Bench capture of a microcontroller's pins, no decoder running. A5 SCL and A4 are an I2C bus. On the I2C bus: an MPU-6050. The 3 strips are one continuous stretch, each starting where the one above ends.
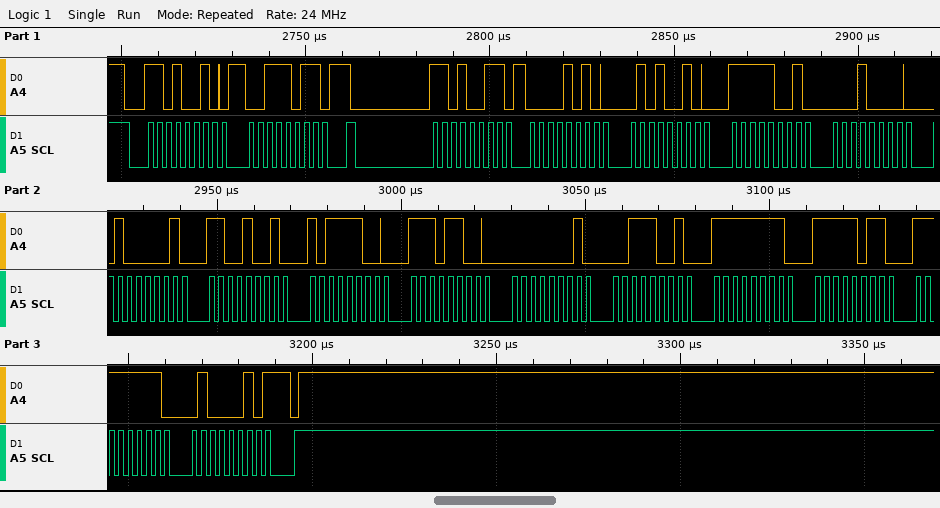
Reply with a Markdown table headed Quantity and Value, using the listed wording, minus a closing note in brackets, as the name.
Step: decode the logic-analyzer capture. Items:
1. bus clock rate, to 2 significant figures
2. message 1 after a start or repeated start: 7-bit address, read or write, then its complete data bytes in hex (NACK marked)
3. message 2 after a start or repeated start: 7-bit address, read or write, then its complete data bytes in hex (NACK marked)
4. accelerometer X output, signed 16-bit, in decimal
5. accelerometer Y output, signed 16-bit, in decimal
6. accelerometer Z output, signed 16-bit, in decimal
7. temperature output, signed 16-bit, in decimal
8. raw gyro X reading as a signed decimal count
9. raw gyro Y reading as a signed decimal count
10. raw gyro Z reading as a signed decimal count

| Quantity | Value |
|---|---|
| bus clock rate, to 2 significant figures | 400 kHz |
| message 1 after a start or repeated start: 7-bit address, read or write, then its complete data bytes in hex | 0x69 write: 3B |
| message 2 after a start or repeated start: 7-bit address, read or write, then its complete data bytes in hex | 0x69 read: 0A 52 F9 10 41 C9 BC EC 01 39 FF FB FF 42 NACK |
| accelerometer X output, signed 16-bit, in decimal | 2642 |
| accelerometer Y output, signed 16-bit, in decimal | -1776 |
| accelerometer Z output, signed 16-bit, in decimal | 16841 |
| temperature output, signed 16-bit, in decimal | -17172 |
| raw gyro X reading as a signed decimal count | 313 |
| raw gyro Y reading as a signed decimal count | -5 |
| raw gyro Z reading as a signed decimal count | -190 |
